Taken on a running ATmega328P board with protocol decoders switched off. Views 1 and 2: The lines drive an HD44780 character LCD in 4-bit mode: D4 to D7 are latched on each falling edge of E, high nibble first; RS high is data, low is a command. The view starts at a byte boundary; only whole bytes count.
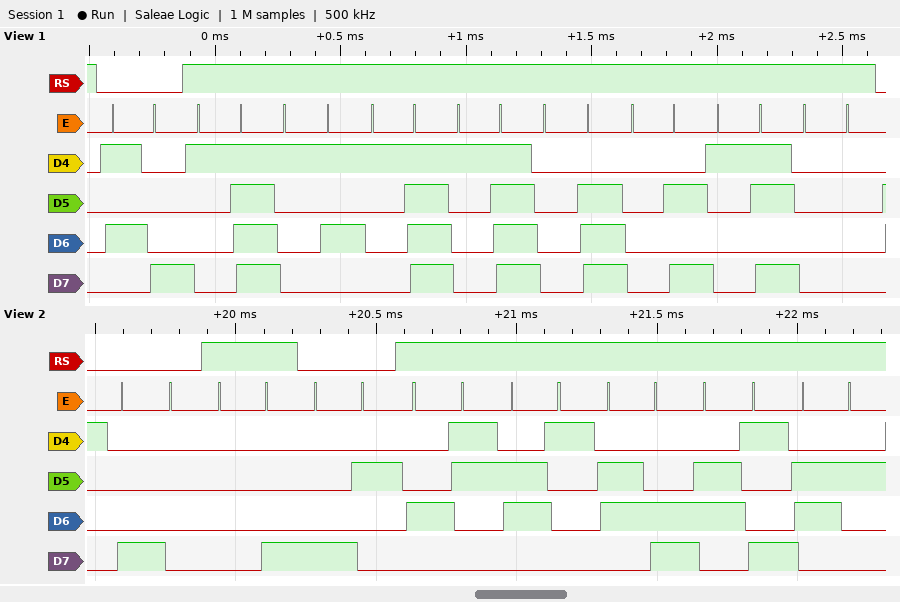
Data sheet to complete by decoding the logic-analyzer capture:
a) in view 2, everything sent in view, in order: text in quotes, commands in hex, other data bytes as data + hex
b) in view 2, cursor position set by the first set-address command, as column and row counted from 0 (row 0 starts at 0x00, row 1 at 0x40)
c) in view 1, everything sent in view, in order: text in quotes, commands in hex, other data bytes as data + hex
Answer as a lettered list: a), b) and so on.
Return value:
a) 0x80 data 08 0x82 "Calib"
b) column 0, row 0
c) 0x58 data 1F 15 1F 1F 0E 0A 1B 00
